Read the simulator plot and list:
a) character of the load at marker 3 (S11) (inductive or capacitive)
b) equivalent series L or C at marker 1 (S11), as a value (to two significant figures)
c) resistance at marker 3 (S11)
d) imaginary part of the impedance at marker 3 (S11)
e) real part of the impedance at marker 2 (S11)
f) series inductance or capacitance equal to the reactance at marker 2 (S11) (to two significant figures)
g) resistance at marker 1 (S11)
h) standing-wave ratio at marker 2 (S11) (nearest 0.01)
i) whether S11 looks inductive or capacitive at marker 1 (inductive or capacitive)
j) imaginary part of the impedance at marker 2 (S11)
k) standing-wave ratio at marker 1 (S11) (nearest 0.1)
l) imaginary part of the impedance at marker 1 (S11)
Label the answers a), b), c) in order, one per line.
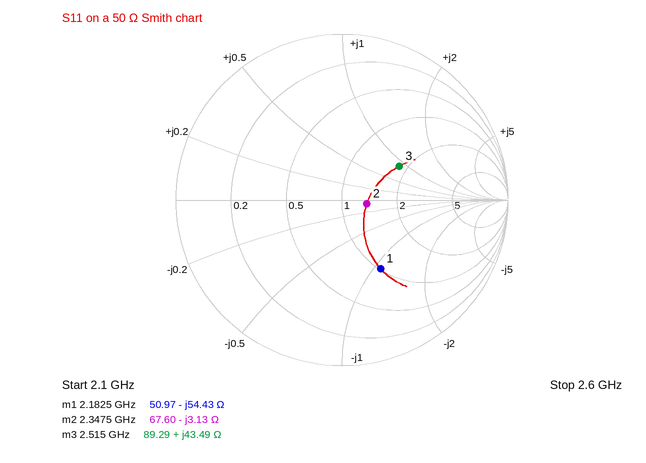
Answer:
a) inductive
b) 1.3 pF
c) 89.29 Ω
d) +43.49 Ω
e) 67.60 Ω
f) 22 pF
g) 50.97 Ω
h) 1.36
i) capacitive
j) -3.13 Ω
k) 2.8
l) -54.43 Ω
